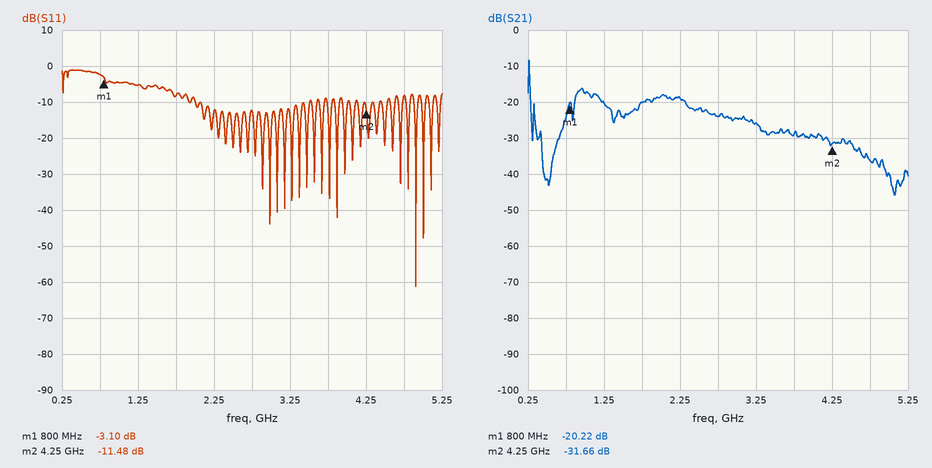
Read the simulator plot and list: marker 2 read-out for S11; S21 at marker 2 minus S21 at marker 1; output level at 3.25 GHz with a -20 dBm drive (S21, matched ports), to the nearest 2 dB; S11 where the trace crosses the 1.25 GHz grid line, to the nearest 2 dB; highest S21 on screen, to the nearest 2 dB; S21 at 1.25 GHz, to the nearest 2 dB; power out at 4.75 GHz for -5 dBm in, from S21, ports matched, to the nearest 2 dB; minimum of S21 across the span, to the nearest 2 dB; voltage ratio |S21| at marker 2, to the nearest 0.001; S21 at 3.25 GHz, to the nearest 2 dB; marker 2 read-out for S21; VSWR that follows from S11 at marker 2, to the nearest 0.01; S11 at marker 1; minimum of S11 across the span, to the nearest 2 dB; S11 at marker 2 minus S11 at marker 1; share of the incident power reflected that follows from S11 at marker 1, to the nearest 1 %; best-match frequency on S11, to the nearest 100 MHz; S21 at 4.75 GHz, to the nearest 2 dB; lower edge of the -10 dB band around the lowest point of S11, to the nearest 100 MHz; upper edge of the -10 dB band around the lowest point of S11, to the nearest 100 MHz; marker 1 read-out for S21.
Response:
-11.48 dB
-11.44 dB
-46 dBm
-6 dB
-8 dB
-20 dB
-42 dBm
-46 dB
0.026
-26 dB
-31.66 dB
1.73
-3.10 dB
-62 dB
-8.38 dB
49 %
4.9 GHz
-36 dB
4.9 GHz
4.9 GHz
-20.22 dB
